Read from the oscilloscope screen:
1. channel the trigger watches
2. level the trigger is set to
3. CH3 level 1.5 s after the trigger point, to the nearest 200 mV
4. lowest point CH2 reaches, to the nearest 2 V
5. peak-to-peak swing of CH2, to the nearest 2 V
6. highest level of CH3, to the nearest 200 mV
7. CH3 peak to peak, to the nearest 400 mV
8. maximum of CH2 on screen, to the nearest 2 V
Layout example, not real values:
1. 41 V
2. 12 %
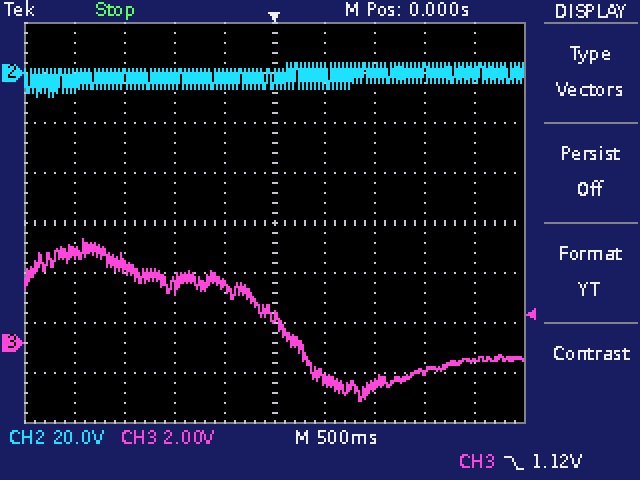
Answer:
1. CH3
2. 1.12 V
3. -1.2 V
4. -10 V
5. 14 V
6. 4.2 V
7. 6.4 V
8. 4 V
